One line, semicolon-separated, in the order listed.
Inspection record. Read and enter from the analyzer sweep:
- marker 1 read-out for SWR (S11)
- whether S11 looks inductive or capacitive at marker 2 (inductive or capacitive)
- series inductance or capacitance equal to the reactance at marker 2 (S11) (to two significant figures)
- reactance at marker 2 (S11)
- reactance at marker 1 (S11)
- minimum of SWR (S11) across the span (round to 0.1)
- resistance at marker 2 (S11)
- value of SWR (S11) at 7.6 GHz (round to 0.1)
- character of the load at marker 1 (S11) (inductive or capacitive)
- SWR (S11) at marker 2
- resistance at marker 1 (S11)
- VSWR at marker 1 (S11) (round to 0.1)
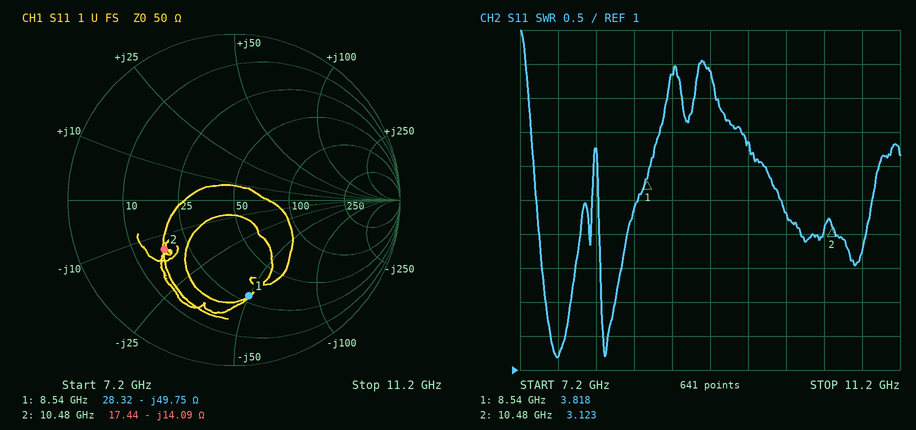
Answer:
3.818; capacitive; 1.1 pF; -14.09 Ω; -49.75 Ω; 1.2; 17.44 Ω; 1.2; capacitive; 3.123; 28.32 Ω; 3.8
